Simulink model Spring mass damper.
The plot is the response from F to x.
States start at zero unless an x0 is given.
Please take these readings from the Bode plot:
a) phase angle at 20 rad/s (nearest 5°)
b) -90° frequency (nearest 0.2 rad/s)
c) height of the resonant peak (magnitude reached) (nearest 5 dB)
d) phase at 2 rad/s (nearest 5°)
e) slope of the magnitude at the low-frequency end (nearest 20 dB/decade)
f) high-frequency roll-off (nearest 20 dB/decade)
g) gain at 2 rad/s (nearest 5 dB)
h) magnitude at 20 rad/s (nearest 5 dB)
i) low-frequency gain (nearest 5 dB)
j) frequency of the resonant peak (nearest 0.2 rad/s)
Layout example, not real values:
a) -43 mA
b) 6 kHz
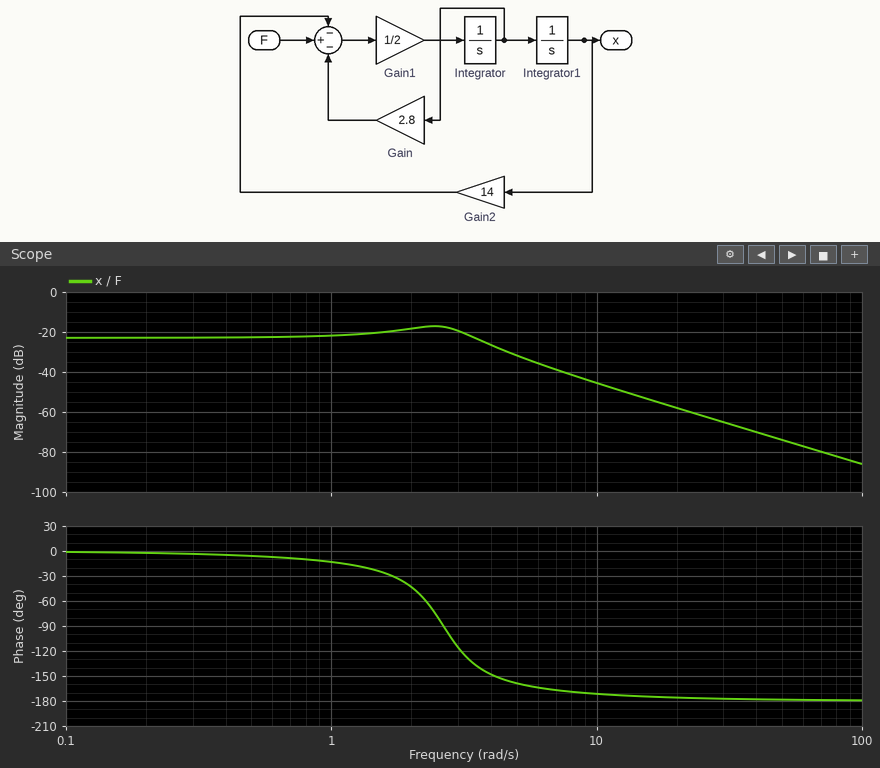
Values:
a) -175°
b) 2.6 rad/s
c) -15 dB
d) -45°
e) 0 dB/decade
f) -40 dB/decade
g) -20 dB
h) -60 dB
i) -25 dB
j) 2.4 rad/s
